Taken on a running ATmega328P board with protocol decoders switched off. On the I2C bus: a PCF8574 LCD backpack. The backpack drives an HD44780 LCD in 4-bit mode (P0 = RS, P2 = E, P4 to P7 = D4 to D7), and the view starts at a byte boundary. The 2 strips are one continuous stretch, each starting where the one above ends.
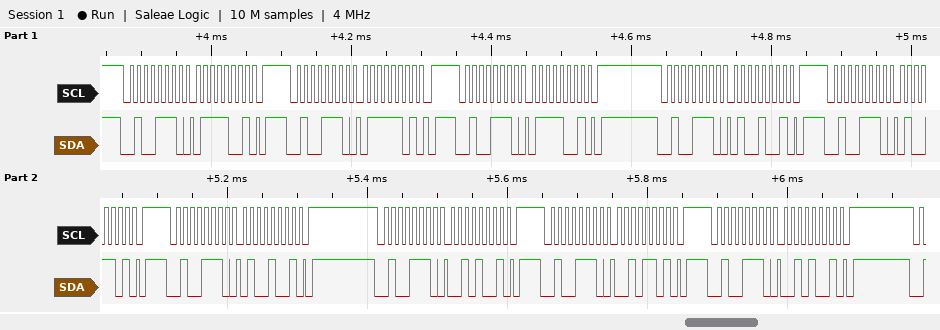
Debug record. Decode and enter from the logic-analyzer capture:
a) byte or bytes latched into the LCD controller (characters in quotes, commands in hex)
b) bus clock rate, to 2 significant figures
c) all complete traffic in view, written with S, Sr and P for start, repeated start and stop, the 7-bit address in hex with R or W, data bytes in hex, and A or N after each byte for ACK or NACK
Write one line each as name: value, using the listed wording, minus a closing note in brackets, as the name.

byte or bytes latched into the LCD controller: 't'
bus clock rate, to 2 significant figures: 100 kHz
all complete traffic in view, written with S, Sr and P for start, repeated start and stop, the 7-bit address in hex with R or W, data bytes in hex, and A or N after each byte for ACK or NACK: S 27W A 79 A P S 27W A 7D A P S 27W A 79 A P S 27W A 49 A P S 27W A 4D A P S 27W A 49 A P S 27W A 29 A P S 27W A 2D A P S 27W A 29 A P
